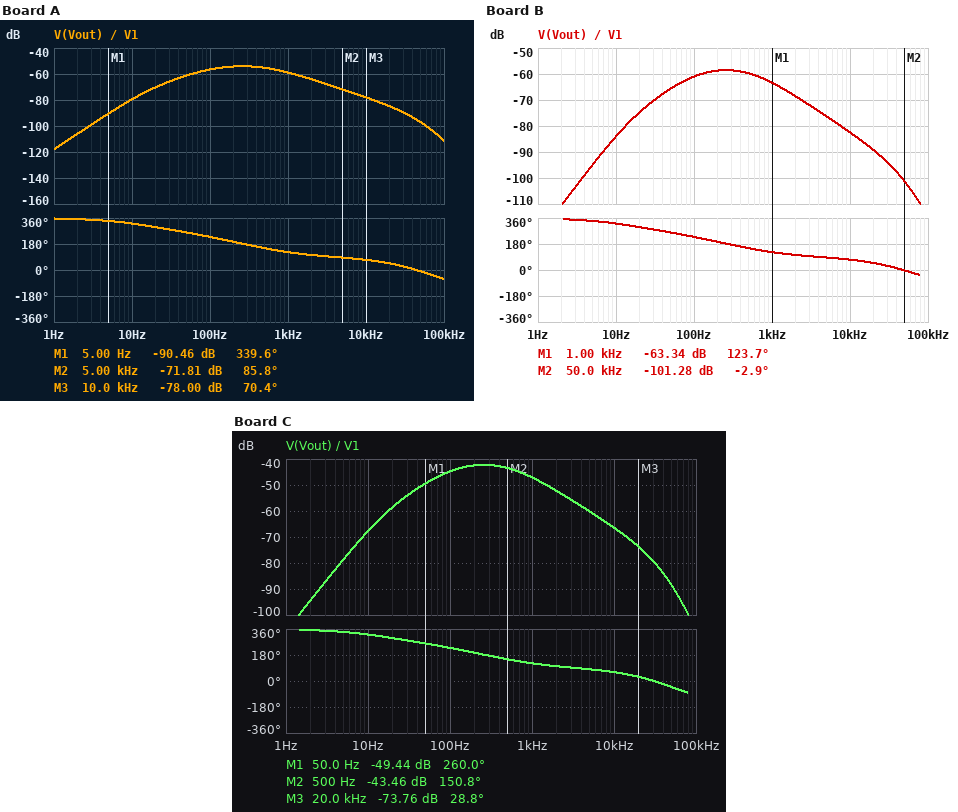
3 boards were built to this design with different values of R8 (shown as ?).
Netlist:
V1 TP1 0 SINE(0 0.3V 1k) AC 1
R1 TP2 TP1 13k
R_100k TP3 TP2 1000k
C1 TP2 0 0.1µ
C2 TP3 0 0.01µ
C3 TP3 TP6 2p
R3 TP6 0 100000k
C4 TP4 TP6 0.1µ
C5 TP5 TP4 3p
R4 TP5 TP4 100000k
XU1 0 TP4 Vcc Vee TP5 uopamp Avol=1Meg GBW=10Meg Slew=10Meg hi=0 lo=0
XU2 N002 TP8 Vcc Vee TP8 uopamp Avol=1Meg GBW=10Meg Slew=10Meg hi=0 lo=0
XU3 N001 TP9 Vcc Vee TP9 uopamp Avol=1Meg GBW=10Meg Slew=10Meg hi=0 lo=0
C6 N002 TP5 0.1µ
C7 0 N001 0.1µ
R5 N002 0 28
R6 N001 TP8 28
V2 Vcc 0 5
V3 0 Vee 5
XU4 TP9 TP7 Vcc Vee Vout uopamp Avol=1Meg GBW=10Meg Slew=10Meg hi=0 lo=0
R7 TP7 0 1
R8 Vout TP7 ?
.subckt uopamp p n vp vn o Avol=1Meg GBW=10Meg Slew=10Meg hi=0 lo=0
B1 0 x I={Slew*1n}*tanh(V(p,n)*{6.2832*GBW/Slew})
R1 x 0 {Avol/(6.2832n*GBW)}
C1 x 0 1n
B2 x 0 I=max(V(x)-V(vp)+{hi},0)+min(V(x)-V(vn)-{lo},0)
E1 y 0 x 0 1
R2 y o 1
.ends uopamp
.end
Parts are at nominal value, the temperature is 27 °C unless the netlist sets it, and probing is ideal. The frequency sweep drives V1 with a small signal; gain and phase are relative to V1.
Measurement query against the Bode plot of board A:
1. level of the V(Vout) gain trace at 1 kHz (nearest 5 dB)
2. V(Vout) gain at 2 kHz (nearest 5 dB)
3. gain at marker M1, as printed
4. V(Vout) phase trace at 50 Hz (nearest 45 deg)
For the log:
-60 dB
-65 dB
-90.46 dB
270 deg
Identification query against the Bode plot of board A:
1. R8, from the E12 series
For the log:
56 Ω
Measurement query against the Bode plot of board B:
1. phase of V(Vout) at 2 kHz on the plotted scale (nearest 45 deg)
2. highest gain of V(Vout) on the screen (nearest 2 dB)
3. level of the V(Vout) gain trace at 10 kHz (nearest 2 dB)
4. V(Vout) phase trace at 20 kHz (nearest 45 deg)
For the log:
90 deg
-58 dB
-82 dB
45 deg
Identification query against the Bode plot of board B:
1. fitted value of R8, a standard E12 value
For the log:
33 Ω
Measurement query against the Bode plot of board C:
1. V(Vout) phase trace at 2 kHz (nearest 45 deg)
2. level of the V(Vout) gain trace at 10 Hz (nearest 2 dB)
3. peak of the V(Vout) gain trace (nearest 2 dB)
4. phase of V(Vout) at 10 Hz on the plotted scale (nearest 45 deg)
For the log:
90 deg
-68 dB
-42 dB
315 deg
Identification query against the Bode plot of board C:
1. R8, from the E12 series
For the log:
220 Ω
